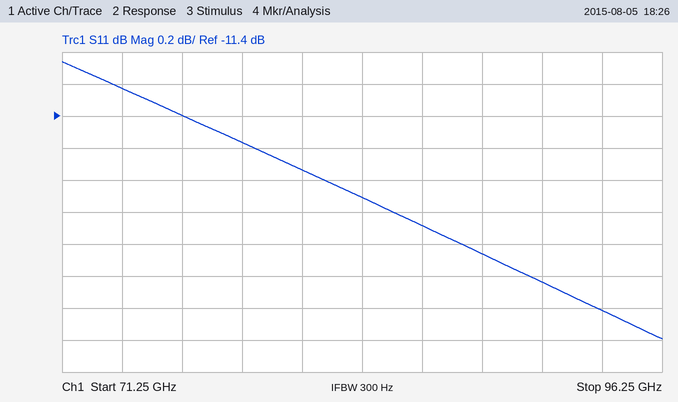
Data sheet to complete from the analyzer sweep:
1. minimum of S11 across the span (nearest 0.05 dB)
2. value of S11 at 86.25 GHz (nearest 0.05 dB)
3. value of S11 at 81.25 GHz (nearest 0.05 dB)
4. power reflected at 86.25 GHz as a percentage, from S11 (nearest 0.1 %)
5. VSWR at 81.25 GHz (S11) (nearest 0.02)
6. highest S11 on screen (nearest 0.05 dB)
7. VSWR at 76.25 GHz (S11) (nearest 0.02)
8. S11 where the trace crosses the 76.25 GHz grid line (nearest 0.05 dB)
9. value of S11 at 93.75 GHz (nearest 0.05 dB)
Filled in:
-12.80 dB
-12.10 dB
-11.75 dB
6.2 %
1.70
-11.05 dB
1.74
-11.40 dB
-12.60 dB
